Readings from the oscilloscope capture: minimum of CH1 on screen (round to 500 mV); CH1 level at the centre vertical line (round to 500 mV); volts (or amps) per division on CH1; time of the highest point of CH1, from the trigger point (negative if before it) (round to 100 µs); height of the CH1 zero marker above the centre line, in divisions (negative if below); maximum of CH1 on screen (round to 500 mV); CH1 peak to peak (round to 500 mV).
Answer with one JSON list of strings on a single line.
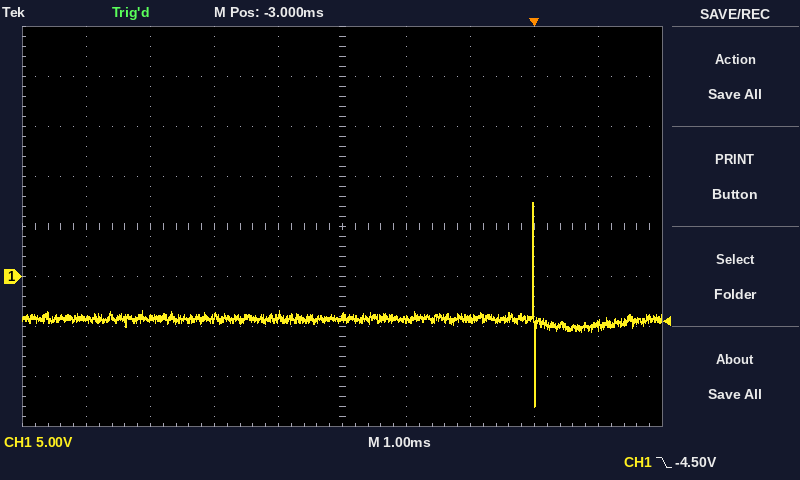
["-13.0 V", "-4.0 V", "5 V", "0.0 ms", "-1.0 div", "7.5 V", "20.5 V"]
